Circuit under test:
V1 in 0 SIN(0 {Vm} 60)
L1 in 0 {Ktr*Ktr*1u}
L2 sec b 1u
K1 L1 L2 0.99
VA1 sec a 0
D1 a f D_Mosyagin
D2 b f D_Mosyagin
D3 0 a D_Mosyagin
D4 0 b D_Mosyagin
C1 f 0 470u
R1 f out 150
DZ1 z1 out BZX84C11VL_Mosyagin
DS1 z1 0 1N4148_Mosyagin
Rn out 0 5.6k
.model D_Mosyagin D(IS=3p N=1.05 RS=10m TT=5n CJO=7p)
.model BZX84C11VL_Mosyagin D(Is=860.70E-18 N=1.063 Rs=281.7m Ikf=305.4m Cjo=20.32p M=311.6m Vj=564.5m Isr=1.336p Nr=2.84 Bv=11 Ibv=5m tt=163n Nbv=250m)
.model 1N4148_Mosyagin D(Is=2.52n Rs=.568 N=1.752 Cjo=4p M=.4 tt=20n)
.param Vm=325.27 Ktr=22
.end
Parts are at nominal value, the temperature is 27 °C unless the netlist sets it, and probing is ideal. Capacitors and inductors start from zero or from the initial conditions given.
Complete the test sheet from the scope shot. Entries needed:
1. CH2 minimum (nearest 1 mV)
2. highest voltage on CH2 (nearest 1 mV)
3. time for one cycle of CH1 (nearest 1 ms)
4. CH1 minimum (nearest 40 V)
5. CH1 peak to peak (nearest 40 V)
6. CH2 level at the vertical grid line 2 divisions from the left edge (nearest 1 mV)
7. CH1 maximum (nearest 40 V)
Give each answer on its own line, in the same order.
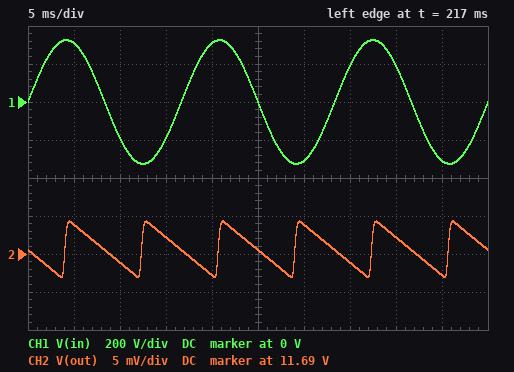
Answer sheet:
11.687 V
11.694 V
17 ms
-320 V
640 V
11.689 V
320 V
